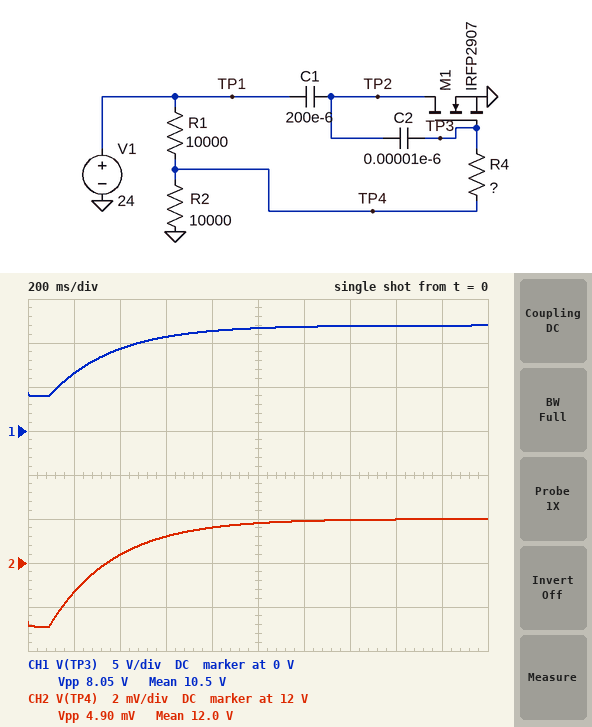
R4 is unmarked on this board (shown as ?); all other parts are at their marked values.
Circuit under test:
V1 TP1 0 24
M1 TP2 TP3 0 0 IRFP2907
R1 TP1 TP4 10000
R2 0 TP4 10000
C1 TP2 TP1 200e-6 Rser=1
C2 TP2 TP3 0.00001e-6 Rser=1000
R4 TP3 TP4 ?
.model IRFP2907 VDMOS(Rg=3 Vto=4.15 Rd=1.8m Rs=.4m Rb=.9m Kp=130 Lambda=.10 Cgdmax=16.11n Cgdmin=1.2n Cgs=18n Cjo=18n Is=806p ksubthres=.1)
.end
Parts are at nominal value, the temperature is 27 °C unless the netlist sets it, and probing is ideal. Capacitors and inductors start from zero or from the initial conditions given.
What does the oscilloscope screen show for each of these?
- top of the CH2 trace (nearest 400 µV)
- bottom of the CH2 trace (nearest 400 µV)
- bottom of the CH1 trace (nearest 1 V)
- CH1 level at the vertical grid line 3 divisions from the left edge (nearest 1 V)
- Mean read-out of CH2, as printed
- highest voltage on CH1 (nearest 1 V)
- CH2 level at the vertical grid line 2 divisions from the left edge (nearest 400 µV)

12.0000 V
11.9952 V
4 V
11 V
12.0 V
12 V
11.9984 V
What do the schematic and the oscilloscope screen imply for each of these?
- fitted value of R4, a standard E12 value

8.2 MΩ
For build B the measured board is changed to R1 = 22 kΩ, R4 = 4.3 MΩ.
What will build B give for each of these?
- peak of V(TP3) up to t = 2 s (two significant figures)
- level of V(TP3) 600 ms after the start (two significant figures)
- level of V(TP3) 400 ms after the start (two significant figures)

7.5 V
7.4 V
7.0 V
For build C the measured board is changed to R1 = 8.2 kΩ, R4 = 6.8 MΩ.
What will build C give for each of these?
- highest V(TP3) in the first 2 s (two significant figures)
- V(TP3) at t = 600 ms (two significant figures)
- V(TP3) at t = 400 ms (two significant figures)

13 V
12 V
11 V
